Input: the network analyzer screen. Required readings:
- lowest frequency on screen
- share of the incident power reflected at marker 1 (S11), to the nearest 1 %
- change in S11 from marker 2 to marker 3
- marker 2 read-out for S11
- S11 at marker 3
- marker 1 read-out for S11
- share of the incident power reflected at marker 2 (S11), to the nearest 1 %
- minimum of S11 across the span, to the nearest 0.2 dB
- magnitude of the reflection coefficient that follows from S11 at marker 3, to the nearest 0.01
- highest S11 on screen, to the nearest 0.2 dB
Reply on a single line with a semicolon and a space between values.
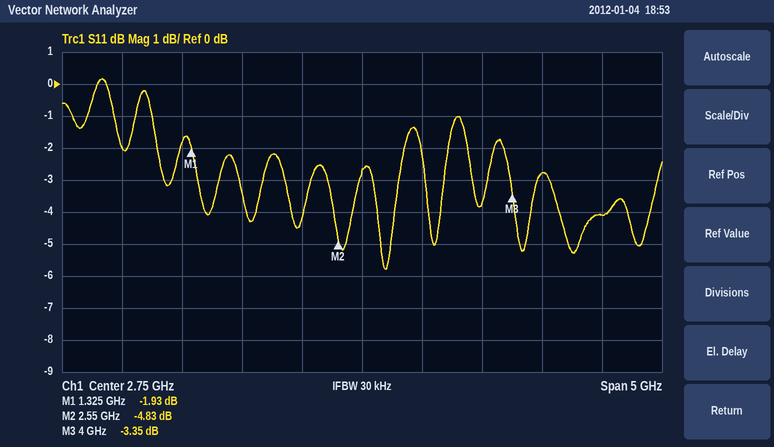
250 MHz; 64 %; 1.48 dB; -4.83 dB; -3.35 dB; -1.93 dB; 33 %; -5.8 dB; 0.68; 0.2 dB
